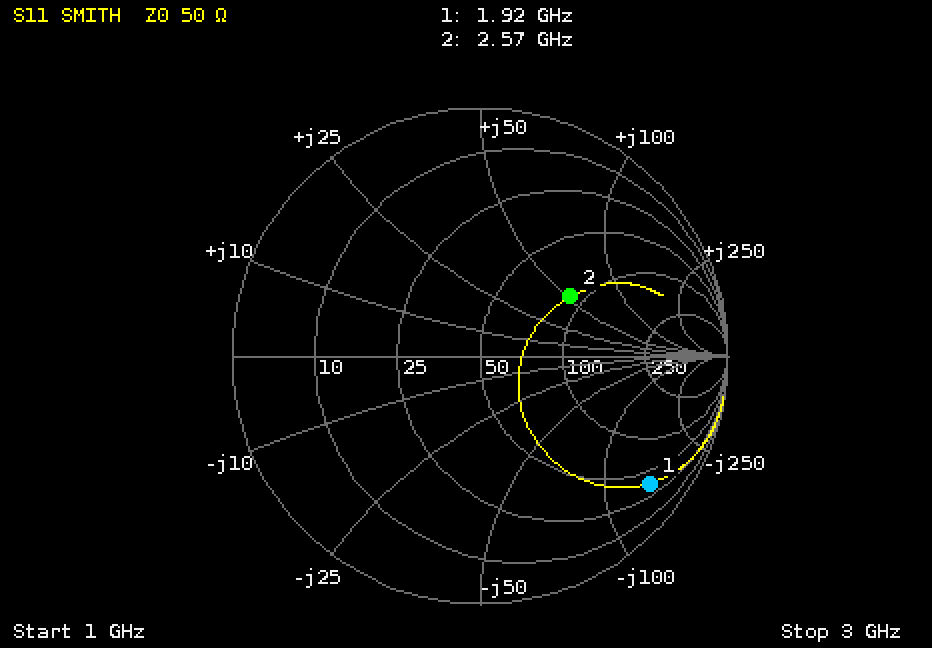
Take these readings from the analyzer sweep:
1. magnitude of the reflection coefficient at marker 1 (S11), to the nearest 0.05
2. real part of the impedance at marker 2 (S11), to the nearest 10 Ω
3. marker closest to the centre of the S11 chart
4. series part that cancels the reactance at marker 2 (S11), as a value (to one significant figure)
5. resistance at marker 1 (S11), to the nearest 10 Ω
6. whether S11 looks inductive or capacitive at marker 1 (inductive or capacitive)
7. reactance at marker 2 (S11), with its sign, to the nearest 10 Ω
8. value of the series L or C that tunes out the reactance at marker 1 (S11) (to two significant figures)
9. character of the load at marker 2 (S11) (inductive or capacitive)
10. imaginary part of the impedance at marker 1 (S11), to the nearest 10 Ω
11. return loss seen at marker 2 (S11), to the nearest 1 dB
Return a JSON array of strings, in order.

["0.85", "90 Ω", "marker 2", "1 pF", "40 Ω", "capacitive", "+50 Ω", "12 nH", "inductive", "-140 Ω", "7 dB"]
